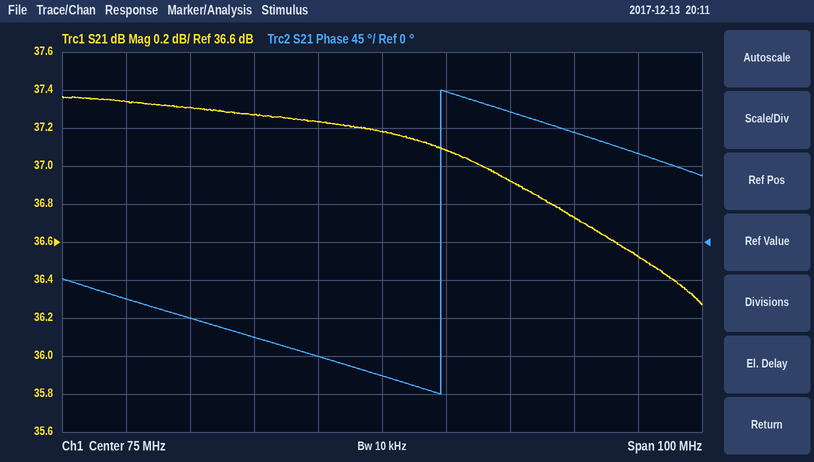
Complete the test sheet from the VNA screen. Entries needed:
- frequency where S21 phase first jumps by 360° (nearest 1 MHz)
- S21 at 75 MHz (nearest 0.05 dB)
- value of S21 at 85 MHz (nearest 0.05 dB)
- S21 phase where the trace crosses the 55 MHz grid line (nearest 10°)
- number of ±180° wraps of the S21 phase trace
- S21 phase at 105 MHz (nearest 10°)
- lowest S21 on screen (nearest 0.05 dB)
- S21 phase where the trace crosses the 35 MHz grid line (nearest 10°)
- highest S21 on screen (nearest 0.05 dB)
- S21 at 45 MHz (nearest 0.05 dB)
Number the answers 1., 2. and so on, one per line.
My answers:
1. 84 MHz
2. 37.20 dB
3. 37.10 dB
4. -110°
5. 1
6. 130°
7. 36.25 dB
8. -70°
9. 37.35 dB
10. 37.30 dB
